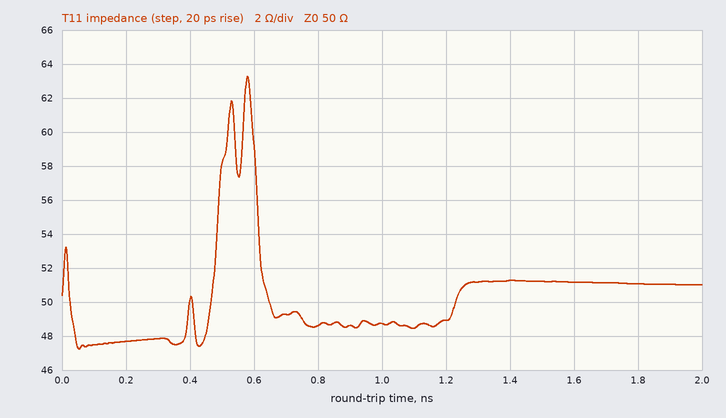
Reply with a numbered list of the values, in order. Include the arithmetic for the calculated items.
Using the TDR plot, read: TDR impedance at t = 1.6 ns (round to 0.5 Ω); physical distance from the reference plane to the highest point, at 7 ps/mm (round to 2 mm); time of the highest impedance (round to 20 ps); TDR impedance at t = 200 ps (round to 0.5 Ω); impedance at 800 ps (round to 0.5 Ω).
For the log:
1. 51.0 Ω
2. 580 ps / 2 / 7 ps/mm ≈ 41.4 mm, so 42 mm to the nearest 2 mm
3. 580 ps
4. 47.5 Ω
5. 48.5 Ω
